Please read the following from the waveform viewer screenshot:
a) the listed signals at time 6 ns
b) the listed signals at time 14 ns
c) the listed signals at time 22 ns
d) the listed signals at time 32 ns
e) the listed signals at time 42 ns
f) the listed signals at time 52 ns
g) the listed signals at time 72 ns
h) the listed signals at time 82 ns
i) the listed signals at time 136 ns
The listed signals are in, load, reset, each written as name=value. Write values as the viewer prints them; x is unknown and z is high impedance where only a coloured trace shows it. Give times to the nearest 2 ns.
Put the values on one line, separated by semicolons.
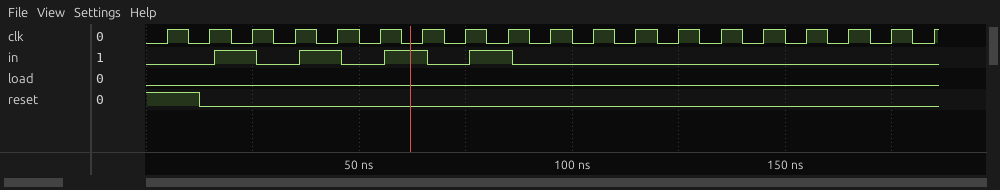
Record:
in=0, load=0, reset=1; in=0, load=0, reset=0; in=1, load=0, reset=0; in=0, load=0, reset=0; in=1, load=0, reset=0; in=0, load=0, reset=0; in=0, load=0, reset=0; in=1, load=0, reset=0; in=0, load=0, reset=0
